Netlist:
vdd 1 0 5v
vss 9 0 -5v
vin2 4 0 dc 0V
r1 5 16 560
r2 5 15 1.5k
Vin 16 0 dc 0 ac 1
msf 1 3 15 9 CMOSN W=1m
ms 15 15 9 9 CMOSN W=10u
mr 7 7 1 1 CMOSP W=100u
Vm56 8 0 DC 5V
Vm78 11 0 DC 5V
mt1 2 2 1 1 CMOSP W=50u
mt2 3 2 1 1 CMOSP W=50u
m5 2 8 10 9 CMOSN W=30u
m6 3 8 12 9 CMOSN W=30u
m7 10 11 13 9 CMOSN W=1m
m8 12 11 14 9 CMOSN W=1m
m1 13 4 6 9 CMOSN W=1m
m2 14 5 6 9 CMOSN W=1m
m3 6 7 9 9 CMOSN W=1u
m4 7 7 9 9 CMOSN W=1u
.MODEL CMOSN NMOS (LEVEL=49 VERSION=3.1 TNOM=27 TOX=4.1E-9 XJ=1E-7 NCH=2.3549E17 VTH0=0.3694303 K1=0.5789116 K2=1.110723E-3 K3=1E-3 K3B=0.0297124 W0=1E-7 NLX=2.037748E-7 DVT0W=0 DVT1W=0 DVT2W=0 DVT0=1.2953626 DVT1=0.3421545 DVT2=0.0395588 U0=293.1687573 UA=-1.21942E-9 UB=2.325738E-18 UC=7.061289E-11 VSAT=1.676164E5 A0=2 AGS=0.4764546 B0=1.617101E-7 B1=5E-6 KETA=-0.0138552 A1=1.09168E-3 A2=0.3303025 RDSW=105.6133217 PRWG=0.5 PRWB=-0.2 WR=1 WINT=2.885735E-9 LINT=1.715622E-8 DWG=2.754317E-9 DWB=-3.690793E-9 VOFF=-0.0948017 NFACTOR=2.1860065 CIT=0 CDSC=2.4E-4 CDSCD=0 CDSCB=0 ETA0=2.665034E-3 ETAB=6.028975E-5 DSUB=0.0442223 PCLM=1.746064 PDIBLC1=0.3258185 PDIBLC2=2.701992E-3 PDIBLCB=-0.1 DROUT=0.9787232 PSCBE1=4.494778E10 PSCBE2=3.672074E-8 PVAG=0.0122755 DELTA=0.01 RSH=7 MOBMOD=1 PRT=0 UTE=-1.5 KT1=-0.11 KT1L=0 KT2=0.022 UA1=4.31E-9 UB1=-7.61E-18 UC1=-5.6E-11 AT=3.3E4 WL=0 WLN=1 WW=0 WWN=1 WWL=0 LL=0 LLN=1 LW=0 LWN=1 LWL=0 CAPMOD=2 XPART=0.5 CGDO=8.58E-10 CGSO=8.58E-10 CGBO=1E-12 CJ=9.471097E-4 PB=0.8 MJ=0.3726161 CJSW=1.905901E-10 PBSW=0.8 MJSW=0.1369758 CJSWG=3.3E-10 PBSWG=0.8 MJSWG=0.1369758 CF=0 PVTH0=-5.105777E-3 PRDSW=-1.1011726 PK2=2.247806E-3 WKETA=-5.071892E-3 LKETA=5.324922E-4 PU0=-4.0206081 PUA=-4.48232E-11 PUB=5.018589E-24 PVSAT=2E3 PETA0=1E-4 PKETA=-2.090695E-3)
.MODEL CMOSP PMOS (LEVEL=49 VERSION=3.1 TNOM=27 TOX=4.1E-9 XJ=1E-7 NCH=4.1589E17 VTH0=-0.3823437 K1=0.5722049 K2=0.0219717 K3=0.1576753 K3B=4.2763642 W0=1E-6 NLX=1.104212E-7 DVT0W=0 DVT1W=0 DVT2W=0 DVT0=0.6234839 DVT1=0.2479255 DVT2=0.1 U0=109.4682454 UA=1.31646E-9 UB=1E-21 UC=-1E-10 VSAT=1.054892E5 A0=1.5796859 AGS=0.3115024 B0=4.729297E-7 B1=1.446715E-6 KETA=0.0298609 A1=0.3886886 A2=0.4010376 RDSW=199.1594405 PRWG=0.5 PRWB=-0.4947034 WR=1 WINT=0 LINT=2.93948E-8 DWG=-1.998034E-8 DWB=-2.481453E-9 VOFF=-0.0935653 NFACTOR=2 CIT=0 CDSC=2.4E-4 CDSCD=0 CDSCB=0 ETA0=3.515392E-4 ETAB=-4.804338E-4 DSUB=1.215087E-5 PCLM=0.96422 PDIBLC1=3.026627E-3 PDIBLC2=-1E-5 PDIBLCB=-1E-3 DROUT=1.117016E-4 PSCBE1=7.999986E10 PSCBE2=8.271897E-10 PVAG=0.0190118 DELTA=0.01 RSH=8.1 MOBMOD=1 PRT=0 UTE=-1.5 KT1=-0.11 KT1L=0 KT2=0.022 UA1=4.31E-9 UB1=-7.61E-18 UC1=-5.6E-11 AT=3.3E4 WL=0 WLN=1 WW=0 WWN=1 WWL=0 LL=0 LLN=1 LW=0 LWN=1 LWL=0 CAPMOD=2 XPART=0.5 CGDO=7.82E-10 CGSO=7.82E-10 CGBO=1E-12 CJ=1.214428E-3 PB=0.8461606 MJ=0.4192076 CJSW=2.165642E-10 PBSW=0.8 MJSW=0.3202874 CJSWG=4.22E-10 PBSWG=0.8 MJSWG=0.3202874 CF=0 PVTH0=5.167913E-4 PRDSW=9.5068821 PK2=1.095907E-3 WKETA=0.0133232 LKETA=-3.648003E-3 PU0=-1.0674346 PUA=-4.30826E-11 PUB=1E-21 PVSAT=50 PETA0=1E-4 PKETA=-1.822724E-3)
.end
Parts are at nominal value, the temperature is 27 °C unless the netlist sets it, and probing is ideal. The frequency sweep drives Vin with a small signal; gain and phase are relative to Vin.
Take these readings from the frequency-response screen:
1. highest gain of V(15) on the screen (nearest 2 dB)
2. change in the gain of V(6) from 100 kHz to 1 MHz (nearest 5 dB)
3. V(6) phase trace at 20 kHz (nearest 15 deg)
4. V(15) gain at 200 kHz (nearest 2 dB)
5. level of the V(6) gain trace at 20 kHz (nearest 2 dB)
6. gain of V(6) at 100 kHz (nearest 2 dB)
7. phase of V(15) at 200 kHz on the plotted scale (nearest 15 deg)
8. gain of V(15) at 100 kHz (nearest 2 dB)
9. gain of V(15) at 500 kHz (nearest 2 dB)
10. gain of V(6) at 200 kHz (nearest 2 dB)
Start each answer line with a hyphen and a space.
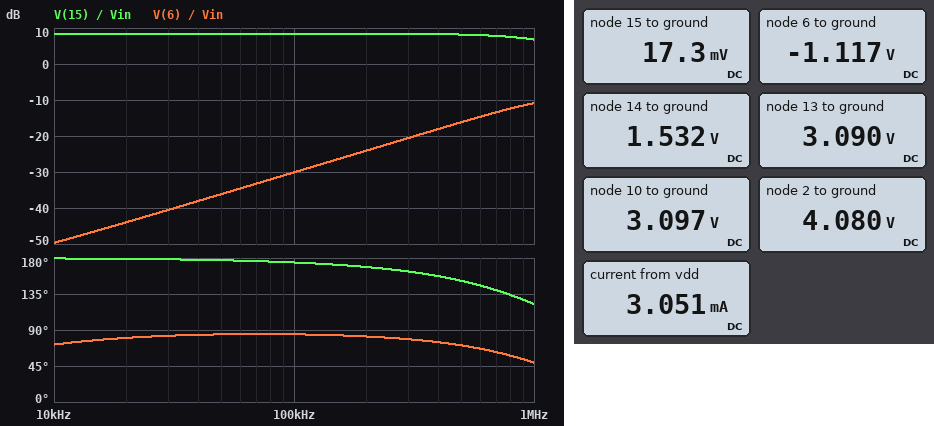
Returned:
- 8 dB
- 20 dB
- 75 deg
- 8 dB
- -44 dB
- -30 dB
- 165 deg
- 8 dB
- 8 dB
- -24 dB
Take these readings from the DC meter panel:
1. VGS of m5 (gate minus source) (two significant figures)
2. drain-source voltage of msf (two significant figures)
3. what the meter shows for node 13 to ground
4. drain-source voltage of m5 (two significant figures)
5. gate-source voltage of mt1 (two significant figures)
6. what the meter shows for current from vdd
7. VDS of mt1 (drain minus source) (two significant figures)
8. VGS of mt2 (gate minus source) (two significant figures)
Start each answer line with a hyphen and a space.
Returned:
- 1.9 V
- 5.0 V
- 3.090 V
- 980 mV
- -920 mV
- 3.051 mA
- -920 mV
- -920 mV
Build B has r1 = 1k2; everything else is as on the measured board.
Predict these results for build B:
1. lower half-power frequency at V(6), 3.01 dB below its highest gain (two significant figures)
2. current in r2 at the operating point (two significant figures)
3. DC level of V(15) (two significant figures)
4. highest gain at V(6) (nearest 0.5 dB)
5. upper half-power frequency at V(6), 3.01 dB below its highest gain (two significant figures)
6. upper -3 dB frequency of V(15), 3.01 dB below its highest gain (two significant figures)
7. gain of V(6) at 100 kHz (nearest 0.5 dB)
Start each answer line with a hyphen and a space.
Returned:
- 1.3 MHz
- 3.9 µA
- 11 mV
- -10.5 dB
- 13 MHz
- 2.1 MHz
- -36.5 dB
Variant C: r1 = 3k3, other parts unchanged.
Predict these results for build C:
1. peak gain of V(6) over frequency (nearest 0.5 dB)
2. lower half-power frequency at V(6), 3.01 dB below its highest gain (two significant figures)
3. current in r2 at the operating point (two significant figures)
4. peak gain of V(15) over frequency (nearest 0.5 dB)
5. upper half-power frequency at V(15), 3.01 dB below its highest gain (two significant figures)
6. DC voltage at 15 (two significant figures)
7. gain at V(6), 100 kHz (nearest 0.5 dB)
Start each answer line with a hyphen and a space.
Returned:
- -14.5 dB
- 1.8 MHz
- 1.4 µA
- -6.0 dB
- 3.3 MHz
- 6.9 mV
- -45.5 dB
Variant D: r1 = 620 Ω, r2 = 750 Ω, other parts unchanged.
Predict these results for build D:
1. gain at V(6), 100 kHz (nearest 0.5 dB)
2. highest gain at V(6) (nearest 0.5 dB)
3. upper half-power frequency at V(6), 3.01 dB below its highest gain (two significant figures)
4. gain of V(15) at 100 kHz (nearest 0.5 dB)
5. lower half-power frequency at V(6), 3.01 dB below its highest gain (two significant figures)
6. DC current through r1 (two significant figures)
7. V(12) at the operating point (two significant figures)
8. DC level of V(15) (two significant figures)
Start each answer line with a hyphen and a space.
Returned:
- -36.5 dB
- -10.5 dB
- 26 MHz
- 1.5 dB
- 1.3 MHz
- 7.6 µA
- 1.5 V
- 10 mV
